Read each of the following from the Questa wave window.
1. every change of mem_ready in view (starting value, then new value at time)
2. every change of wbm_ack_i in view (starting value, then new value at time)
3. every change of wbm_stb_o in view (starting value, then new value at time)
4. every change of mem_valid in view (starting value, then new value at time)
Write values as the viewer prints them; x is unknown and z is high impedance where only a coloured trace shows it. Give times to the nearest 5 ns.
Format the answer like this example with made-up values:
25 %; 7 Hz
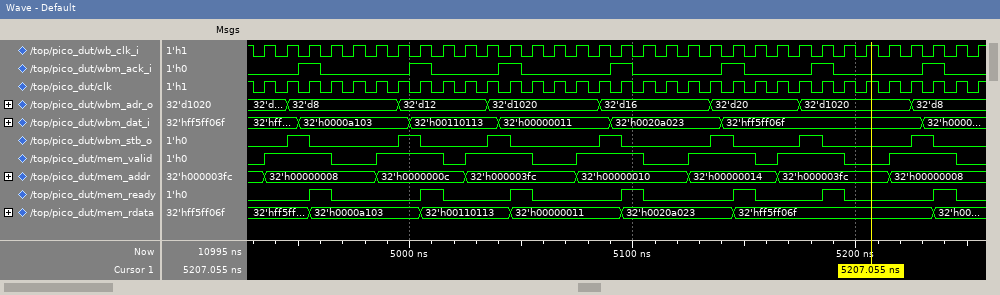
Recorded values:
0, 1 at 4955 ns, 0 at 4965 ns, 1 at 5005 ns, 0 at 5015 ns, 1 at 5045 ns, 0 at 5055 ns, 1 at 5095 ns, 0 at 5105 ns, 1 at 5145 ns, 0 at 5155 ns, 1 at 5185 ns, 0 at 5195 ns, 1 at 5235 ns, 0 at 5245 ns; 0, 1 at 4950 ns, 0 at 4960 ns, 1 at 5000 ns, 0 at 5010 ns, 1 at 5040 ns, 0 at 5050 ns, 1 at 5090 ns, 0 at 5100 ns, 1 at 5140 ns, 0 at 5150 ns, 1 at 5180 ns, 0 at 5190 ns, 1 at 5230 ns, 0 at 5240 ns; 0, 1 at 4945 ns, 0 at 4955 ns, 1 at 4995 ns, 0 at 5005 ns, 1 at 5035 ns, 0 at 5045 ns, 1 at 5085 ns, 0 at 5095 ns, 1 at 5135 ns, 0 at 5145 ns, 1 at 5175 ns, 0 at 5185 ns, 1 at 5225 ns, 0 at 5235 ns; 0, 1 at 4935 ns, 0 at 4965 ns, 1 at 4985 ns, 0 at 5015 ns, 1 at 5025 ns, 0 at 5055 ns, 1 at 5075 ns, 0 at 5105 ns, 1 at 5125 ns, 0 at 5155 ns, 1 at 5165 ns, 0 at 5195 ns, 1 at 5215 ns, 0 at 5245 ns
